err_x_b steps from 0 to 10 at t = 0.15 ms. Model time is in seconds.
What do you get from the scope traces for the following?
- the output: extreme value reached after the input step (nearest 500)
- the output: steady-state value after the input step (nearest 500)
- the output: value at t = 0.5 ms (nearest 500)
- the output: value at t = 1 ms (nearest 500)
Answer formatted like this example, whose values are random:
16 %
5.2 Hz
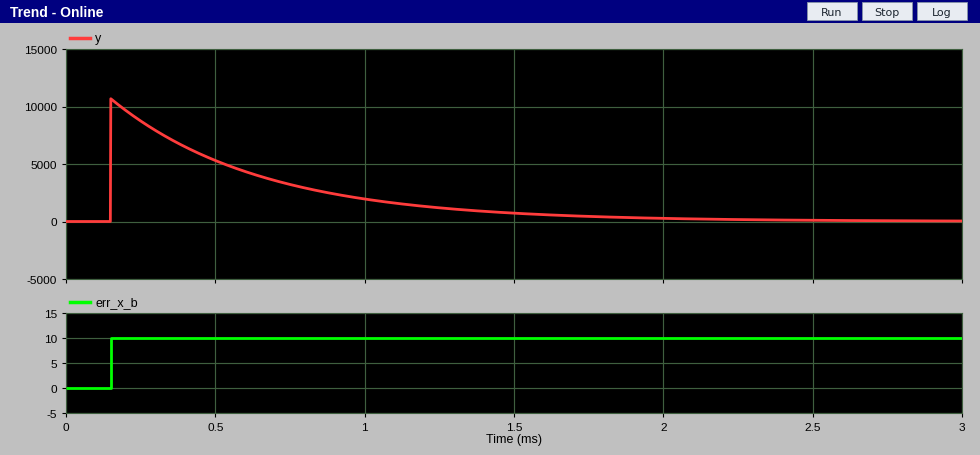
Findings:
10500
0
5500
2000
